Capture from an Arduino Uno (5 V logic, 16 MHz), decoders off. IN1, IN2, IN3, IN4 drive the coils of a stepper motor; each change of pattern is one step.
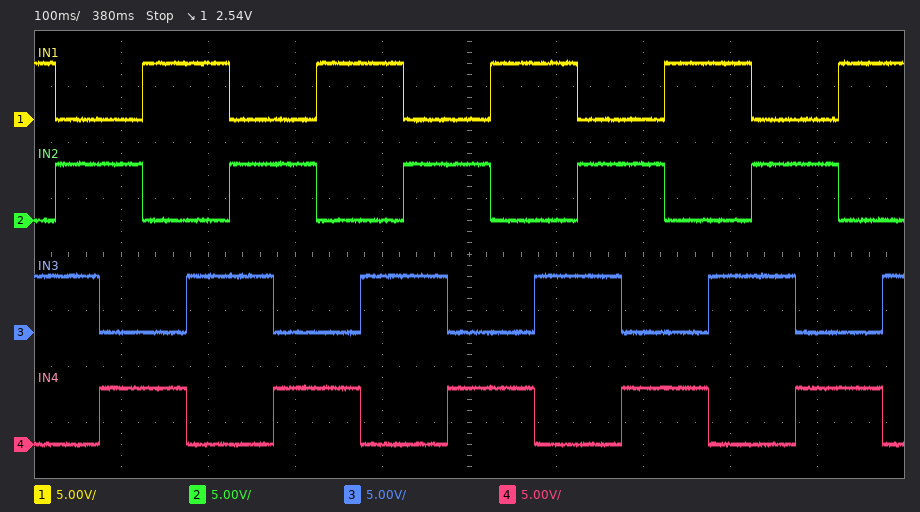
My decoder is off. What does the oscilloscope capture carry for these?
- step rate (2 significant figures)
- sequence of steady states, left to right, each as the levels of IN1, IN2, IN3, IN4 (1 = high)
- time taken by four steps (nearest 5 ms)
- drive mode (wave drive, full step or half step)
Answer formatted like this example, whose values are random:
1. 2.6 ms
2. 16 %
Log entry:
1. 20 steps/s
2. 1010 0110 0101 1001 1010 0110 0101 1001 1010 0110 0101 1001 1010 0110 0101 1001 1010 0110 0101 1001 1010
3. 200 ms
4. full step
